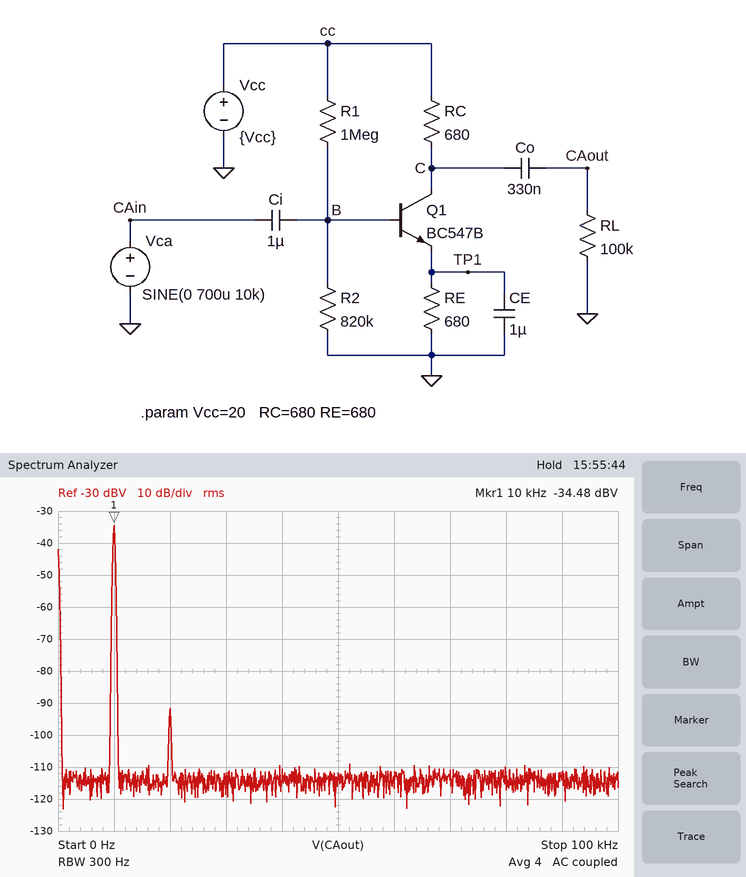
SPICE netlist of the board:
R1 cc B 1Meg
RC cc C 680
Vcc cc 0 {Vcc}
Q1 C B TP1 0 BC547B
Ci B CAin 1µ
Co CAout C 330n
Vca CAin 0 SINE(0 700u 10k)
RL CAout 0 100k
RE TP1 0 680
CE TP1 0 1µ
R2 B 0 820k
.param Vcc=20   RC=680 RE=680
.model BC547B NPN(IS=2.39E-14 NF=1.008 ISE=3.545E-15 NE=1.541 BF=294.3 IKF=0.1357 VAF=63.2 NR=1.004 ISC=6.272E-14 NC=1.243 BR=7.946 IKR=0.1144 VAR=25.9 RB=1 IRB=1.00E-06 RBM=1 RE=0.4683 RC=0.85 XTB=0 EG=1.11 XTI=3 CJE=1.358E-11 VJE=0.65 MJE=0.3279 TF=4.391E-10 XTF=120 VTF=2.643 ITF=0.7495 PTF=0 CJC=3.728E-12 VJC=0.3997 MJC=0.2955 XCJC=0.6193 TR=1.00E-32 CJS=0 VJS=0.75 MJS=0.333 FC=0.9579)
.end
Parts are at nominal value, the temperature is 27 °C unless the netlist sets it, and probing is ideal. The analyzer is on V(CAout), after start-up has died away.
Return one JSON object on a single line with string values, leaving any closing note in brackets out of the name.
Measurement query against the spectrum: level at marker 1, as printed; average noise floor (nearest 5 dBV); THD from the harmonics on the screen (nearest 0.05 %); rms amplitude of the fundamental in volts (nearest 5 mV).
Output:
{"level at marker 1, as printed": "-34.48 dBV", "average noise floor": "-115 dBV", "THD from the harmonics on the screen": "0.15 %", "rms amplitude of the fundamental in volts": "20 mV"}
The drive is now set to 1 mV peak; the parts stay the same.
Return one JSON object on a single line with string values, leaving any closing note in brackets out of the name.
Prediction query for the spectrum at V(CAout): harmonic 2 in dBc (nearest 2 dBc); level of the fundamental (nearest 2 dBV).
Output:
{"harmonic 2 in dBc": "-54 dBc", "level of the fundamental": "-32 dBV"}
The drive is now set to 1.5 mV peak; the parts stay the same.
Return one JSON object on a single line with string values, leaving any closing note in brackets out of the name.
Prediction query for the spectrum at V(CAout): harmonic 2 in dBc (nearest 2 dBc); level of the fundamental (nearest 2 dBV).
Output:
{"harmonic 2 in dBc": "-50 dBc", "level of the fundamental": "-28 dBV"}
